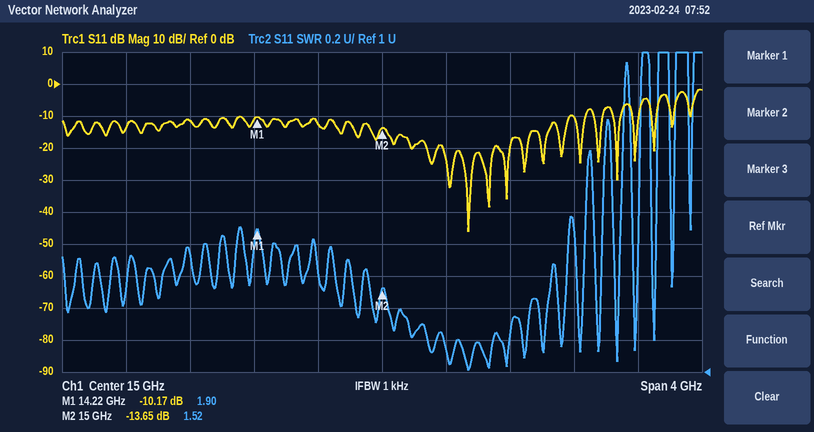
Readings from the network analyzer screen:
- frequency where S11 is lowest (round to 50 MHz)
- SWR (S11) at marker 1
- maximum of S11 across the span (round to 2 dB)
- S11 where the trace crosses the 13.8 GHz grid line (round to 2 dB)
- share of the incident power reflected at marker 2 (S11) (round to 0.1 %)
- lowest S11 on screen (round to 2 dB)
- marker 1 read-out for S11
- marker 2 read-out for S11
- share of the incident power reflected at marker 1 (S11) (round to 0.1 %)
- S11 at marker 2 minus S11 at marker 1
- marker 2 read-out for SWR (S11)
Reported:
15.55 GHz
1.90
-2 dB
-12 dB
4.3 %
-46 dB
-10.17 dB
-13.65 dB
9.6 %
-3.48 dB
1.52
